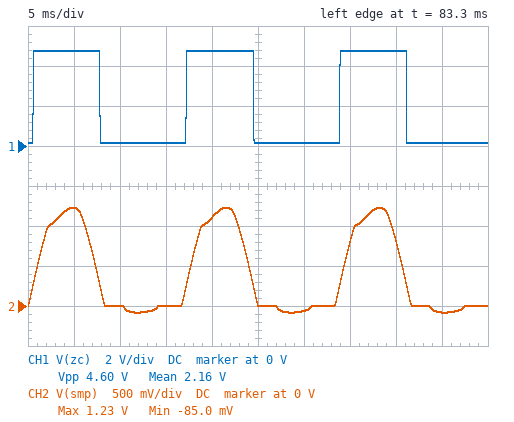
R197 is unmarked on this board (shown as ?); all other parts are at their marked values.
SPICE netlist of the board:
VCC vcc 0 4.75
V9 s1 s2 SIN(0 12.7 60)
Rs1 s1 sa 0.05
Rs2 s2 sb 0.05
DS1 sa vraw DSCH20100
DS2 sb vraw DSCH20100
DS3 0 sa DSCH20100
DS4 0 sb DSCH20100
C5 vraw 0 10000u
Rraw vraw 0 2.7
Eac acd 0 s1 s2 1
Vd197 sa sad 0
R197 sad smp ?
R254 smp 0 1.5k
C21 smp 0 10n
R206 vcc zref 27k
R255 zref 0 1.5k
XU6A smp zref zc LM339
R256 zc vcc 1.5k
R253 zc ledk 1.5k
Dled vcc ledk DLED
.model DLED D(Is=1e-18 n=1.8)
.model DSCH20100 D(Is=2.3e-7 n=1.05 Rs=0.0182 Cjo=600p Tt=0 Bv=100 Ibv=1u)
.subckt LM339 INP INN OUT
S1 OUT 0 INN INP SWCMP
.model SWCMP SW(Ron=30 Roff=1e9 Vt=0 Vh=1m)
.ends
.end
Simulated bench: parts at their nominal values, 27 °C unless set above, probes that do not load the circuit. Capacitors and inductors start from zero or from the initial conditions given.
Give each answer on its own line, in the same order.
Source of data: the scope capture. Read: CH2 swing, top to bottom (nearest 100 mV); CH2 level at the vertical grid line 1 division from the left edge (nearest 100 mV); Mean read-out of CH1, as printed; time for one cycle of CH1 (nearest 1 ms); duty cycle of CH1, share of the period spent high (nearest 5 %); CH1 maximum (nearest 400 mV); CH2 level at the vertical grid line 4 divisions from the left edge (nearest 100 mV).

1.3 V
1.2 V
2.16 V
17 ms
45 %
4.8 V
1.1 V
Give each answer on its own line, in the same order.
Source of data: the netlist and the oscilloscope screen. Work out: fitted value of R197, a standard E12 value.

12 kΩ
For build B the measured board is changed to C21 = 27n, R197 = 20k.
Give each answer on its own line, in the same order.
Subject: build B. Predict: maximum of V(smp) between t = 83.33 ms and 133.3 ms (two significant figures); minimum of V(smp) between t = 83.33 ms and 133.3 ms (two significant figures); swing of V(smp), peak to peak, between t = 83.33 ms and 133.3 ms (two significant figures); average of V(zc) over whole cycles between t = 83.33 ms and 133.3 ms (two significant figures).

770 mV
-52 mV
820 mV
2.0 V
